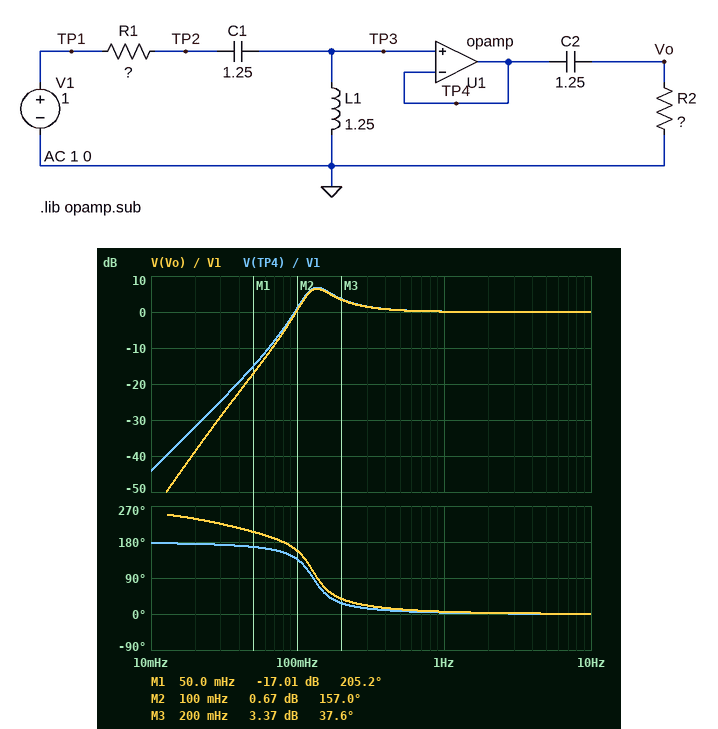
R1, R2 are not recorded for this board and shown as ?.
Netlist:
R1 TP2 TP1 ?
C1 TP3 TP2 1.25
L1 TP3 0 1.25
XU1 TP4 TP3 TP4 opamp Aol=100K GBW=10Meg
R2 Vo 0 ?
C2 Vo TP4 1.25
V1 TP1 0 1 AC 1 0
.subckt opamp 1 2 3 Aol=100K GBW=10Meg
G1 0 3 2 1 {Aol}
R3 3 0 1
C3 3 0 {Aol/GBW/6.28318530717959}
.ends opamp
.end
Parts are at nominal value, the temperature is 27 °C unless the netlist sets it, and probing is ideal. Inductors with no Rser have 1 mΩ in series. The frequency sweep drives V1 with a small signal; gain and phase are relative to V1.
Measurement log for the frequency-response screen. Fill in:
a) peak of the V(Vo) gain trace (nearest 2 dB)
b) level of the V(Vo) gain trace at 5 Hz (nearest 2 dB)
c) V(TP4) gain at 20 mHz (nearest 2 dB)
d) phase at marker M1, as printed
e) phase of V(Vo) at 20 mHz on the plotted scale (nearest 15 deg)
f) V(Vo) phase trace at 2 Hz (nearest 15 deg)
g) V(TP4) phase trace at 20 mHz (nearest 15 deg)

6 dB
0 dB
-32 dB
205.2 deg
240 deg
0 deg
180 deg
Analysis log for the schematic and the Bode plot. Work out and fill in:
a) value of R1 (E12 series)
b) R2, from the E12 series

0.47 Ω
3.3 Ω
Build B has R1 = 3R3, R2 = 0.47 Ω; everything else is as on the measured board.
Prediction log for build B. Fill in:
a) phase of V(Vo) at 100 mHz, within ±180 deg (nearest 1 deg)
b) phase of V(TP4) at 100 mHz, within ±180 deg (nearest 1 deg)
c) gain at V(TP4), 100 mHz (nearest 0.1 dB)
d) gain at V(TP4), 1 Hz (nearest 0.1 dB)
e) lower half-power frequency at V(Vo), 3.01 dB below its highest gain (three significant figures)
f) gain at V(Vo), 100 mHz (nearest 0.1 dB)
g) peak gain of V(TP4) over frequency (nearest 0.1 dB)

168 deg
98 deg
-12.6 dB
-0.6 dB
510 mHz
-21.8 dB
0 dB
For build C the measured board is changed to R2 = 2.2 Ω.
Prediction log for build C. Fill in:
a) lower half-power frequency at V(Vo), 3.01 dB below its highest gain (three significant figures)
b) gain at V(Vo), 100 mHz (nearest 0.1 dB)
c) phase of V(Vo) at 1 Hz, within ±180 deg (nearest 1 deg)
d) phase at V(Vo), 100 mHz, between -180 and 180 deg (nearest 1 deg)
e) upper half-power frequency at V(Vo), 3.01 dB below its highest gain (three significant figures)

111 mHz
0 dB
7 deg
166 deg
204 mHz
